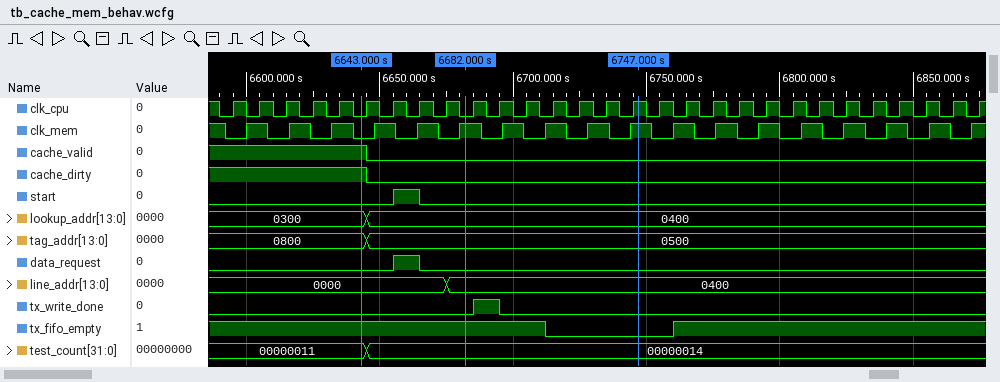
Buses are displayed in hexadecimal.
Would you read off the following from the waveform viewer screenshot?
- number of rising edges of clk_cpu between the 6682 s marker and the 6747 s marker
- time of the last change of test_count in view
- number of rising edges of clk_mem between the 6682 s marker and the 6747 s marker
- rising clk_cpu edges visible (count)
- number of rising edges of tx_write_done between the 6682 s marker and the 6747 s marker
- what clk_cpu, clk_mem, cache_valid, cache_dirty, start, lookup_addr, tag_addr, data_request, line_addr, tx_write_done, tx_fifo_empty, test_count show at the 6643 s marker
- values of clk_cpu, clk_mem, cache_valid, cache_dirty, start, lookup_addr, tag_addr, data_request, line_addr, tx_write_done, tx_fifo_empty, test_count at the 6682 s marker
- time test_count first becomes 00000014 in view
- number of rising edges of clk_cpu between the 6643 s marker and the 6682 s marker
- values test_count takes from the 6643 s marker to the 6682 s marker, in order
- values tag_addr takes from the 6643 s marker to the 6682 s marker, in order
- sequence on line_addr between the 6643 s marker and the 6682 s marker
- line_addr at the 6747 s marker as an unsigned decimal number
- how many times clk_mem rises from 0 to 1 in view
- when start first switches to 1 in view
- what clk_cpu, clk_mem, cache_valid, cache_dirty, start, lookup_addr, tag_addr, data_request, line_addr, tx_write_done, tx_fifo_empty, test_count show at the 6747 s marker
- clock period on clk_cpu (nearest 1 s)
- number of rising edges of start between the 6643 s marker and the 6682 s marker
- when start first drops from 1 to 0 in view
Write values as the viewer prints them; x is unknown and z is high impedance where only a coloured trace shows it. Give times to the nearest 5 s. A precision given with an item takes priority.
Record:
7
6645 s
4
29
1
clk_cpu=0, clk_mem=0, cache_valid=1, cache_dirty=1, start=0, lookup_addr=0300, tag_addr=0800, data_request=0, line_addr=0000, tx_write_done=0, tx_fifo_empty=1, test_count=00000011
clk_cpu=0, clk_mem=1, cache_valid=0, cache_dirty=0, start=0, lookup_addr=0400, tag_addr=0500, data_request=0, line_addr=0400, tx_write_done=0, tx_fifo_empty=1, test_count=00000014
6645 s
4
00000011, 00000014
0800, 0500
0000, 0400
1024
18
6655 s
clk_cpu=1, clk_mem=1, cache_valid=0, cache_dirty=0, start=0, lookup_addr=0400, tag_addr=0500, data_request=0, line_addr=0400, tx_write_done=0, tx_fifo_empty=0, test_count=00000014
10 s
1
6665 s
